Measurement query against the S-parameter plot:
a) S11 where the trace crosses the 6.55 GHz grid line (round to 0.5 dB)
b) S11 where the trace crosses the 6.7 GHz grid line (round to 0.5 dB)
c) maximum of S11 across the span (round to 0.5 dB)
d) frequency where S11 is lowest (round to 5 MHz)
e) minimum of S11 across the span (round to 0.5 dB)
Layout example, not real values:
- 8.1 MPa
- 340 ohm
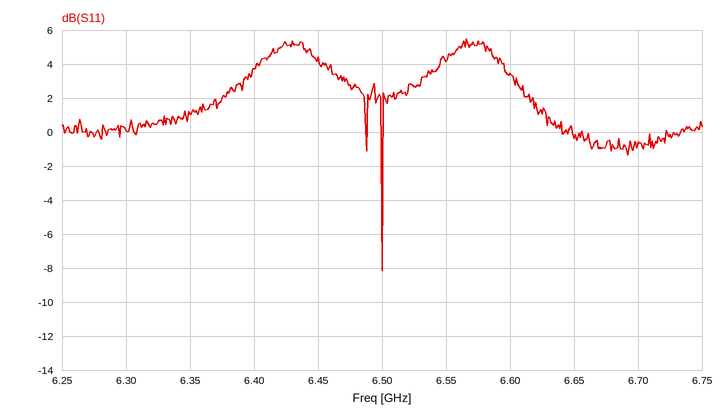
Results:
- 4.0 dB
- -0.5 dB
- 5.5 dB
- 6.500 GHz
- -8.0 dB
